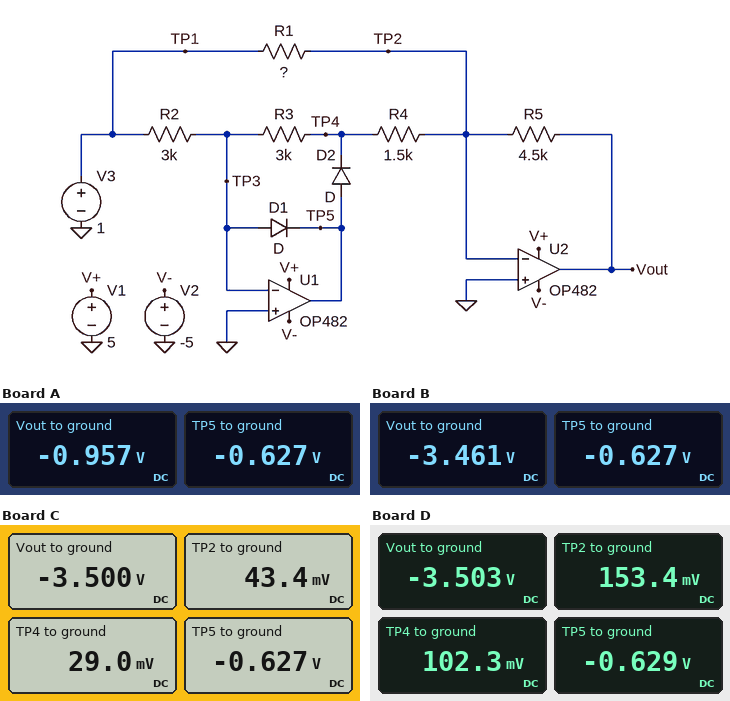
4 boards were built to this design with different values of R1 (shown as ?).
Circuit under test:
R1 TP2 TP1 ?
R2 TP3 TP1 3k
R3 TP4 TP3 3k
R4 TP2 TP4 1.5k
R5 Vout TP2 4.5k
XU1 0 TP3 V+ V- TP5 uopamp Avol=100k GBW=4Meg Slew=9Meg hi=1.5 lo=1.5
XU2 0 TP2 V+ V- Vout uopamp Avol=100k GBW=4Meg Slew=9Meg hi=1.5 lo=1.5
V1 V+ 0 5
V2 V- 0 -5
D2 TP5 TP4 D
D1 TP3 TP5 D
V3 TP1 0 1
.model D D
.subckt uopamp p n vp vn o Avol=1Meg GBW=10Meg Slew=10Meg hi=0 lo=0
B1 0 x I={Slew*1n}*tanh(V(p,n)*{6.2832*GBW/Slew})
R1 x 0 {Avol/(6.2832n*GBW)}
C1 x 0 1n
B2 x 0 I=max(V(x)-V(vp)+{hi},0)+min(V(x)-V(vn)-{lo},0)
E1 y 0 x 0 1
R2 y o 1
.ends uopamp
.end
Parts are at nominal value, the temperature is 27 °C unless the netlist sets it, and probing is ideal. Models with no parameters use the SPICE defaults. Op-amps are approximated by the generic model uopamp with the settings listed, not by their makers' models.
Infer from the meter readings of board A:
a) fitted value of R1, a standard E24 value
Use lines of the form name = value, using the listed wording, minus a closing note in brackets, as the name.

fitted value of R1, a standard E24 value = 4.7 kΩ
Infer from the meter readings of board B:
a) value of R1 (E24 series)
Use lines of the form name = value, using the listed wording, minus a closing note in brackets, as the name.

value of R1 = 1.3 kΩ
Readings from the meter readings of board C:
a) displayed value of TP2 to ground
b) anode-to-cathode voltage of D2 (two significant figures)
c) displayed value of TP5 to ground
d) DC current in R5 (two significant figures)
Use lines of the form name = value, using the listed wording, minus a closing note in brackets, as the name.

displayed value of TP2 to ground = 43.4 mV
anode-to-cathode voltage of D2 = -660 mV
displayed value of TP5 to ground = -0.627 V
DC current in R5 = 790 µA
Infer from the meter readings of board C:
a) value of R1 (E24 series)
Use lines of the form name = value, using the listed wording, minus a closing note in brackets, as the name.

value of R1 = 1.2 kΩ
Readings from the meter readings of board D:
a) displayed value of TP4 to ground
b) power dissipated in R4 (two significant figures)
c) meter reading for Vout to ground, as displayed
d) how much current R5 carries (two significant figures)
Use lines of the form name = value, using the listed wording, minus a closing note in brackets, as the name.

displayed value of TP4 to ground = 102.3 mV
power dissipated in R4 = 1.7 µW
meter reading for Vout to ground, as displayed = -3.503 V
how much current R5 carries = 810 µA
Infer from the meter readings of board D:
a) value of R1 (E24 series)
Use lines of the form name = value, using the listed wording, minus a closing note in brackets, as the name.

value of R1 = 1 kΩ
